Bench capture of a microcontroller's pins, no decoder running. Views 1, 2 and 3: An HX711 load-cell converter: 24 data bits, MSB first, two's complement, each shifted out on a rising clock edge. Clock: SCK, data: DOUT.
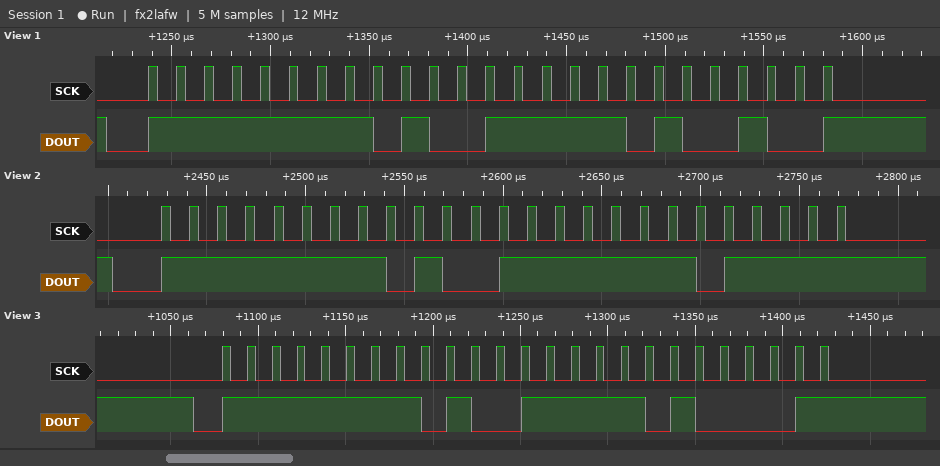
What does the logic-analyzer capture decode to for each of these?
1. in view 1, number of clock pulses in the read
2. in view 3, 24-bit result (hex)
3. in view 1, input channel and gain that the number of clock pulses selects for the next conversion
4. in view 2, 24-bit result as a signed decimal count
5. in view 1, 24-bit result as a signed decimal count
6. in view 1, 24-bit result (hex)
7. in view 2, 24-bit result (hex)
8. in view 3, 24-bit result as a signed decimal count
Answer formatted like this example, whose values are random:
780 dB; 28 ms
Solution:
25; 0xFF4FA1; channel A, gain 128; -45073; -45148; 0xFF4FA4; 0xFF4FEF; -45151
